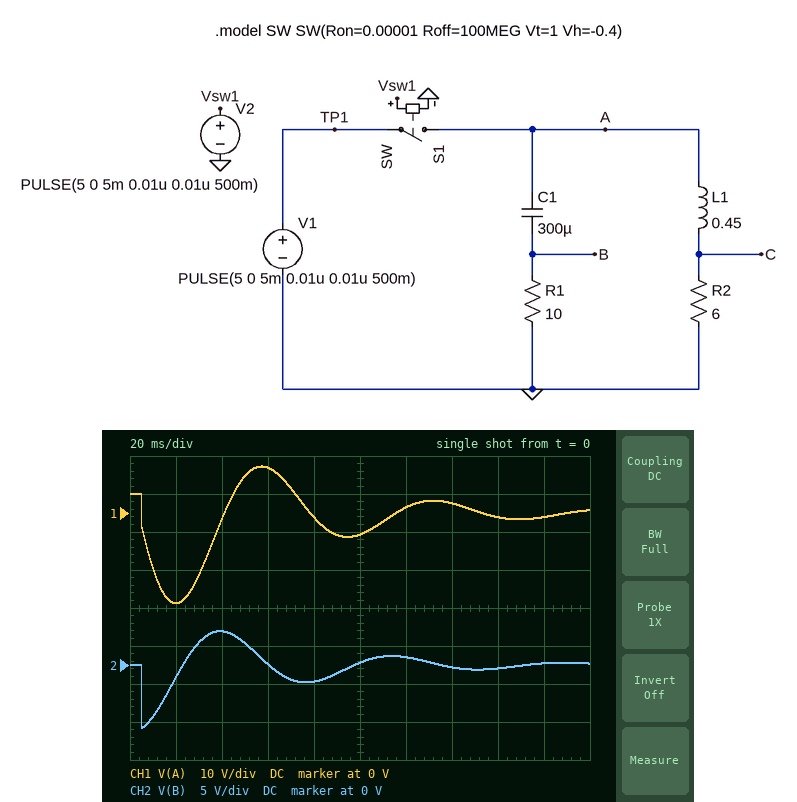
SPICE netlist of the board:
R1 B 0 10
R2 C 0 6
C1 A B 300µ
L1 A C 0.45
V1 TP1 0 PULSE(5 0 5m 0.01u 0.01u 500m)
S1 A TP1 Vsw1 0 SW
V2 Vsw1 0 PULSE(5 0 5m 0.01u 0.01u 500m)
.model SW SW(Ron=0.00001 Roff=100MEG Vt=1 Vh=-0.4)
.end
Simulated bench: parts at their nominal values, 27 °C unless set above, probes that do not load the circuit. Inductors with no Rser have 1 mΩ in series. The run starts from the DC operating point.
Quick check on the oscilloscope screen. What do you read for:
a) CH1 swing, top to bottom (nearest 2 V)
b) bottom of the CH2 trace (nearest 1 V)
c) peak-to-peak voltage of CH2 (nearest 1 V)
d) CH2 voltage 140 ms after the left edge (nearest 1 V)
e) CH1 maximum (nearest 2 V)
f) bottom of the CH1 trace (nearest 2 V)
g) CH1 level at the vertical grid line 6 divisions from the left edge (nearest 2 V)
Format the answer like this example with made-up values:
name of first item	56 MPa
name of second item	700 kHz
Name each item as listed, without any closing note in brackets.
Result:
CH1 swing, top to bottom	36 V
bottom of the CH2 trace	-8 V
peak-to-peak voltage of CH2	13 V
CH2 voltage 140 ms after the left edge	0 V
CH1 maximum	12 V
bottom of the CH1 trace	-24 V
CH1 level at the vertical grid line 6 divisions from the left edge	2 V
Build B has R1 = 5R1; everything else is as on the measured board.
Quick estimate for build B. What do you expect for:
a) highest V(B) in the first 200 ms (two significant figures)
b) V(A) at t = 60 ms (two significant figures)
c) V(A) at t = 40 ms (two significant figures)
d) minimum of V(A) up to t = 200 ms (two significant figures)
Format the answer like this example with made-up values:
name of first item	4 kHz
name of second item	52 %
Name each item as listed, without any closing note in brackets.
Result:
highest V(B) in the first 200 ms	2.7 V
V(A) at t = 60 ms	16 V
V(A) at t = 40 ms	-3.8 V
minimum of V(A) up to t = 200 ms	-26 V
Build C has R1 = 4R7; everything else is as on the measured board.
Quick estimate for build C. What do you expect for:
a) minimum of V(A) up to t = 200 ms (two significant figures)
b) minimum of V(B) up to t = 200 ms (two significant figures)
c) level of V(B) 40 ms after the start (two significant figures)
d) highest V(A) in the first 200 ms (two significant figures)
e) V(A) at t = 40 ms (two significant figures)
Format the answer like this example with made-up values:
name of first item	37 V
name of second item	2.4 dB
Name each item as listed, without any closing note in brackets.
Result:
minimum of V(A) up to t = 200 ms	-26 V
minimum of V(B) up to t = 200 ms	-3.9 V
level of V(B) 40 ms after the start	2.5 V
highest V(A) in the first 200 ms	17 V
V(A) at t = 40 ms	-4.0 V
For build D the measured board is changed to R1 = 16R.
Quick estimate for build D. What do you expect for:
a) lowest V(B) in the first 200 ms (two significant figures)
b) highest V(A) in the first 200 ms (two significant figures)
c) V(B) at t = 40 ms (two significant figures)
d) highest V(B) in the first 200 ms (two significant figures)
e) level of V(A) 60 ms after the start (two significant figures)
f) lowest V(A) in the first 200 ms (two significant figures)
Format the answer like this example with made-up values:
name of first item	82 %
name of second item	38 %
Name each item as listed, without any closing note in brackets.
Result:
lowest V(B) in the first 200 ms	-13 V
highest V(A) in the first 200 ms	8.8 V
V(B) at t = 40 ms	5.7 V
highest V(B) in the first 200 ms	5.8 V
level of V(A) 60 ms after the start	8.2 V
lowest V(A) in the first 200 ms	-22 V
